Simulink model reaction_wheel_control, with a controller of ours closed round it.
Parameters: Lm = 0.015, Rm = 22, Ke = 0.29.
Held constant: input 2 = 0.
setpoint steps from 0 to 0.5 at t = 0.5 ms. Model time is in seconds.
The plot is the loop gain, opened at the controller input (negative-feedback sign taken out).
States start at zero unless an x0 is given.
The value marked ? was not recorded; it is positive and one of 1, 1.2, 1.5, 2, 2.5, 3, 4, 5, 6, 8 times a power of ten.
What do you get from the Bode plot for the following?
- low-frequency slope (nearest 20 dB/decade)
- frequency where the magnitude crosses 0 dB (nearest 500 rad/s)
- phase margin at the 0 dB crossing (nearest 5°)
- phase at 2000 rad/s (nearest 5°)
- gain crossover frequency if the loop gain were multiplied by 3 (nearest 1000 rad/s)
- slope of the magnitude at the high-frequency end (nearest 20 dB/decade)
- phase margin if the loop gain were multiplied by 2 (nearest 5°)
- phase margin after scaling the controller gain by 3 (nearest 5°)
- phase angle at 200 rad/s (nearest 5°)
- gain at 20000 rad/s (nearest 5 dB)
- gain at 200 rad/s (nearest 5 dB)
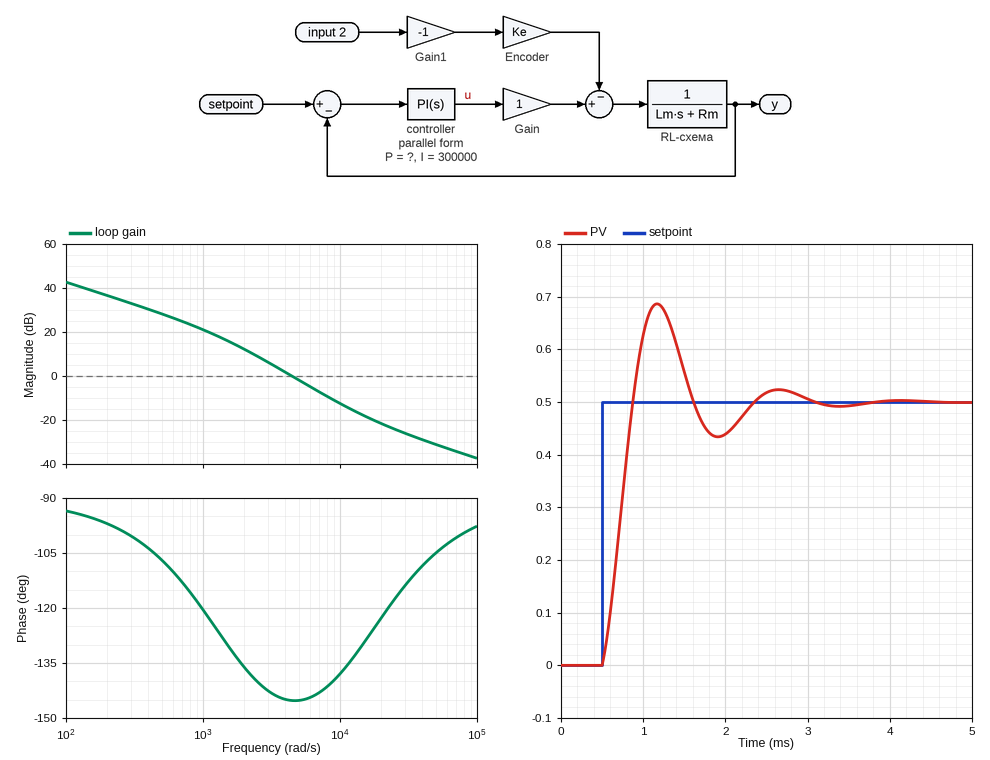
-20 dB/decade
4500 rad/s
35°
-135°
8000 rad/s
-20 dB/decade
35°
40°
-95°
-20 dB
35 dB
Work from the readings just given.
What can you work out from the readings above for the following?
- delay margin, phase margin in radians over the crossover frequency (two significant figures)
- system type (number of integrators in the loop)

0.00014 s
1
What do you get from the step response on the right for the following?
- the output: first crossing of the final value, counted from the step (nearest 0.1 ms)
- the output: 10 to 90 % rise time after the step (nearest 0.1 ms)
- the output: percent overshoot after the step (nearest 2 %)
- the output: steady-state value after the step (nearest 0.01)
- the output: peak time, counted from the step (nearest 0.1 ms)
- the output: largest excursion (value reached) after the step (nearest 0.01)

0.4 ms
0.3 ms
38 %
0.50
0.7 ms
0.69
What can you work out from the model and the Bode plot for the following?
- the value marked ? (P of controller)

20
